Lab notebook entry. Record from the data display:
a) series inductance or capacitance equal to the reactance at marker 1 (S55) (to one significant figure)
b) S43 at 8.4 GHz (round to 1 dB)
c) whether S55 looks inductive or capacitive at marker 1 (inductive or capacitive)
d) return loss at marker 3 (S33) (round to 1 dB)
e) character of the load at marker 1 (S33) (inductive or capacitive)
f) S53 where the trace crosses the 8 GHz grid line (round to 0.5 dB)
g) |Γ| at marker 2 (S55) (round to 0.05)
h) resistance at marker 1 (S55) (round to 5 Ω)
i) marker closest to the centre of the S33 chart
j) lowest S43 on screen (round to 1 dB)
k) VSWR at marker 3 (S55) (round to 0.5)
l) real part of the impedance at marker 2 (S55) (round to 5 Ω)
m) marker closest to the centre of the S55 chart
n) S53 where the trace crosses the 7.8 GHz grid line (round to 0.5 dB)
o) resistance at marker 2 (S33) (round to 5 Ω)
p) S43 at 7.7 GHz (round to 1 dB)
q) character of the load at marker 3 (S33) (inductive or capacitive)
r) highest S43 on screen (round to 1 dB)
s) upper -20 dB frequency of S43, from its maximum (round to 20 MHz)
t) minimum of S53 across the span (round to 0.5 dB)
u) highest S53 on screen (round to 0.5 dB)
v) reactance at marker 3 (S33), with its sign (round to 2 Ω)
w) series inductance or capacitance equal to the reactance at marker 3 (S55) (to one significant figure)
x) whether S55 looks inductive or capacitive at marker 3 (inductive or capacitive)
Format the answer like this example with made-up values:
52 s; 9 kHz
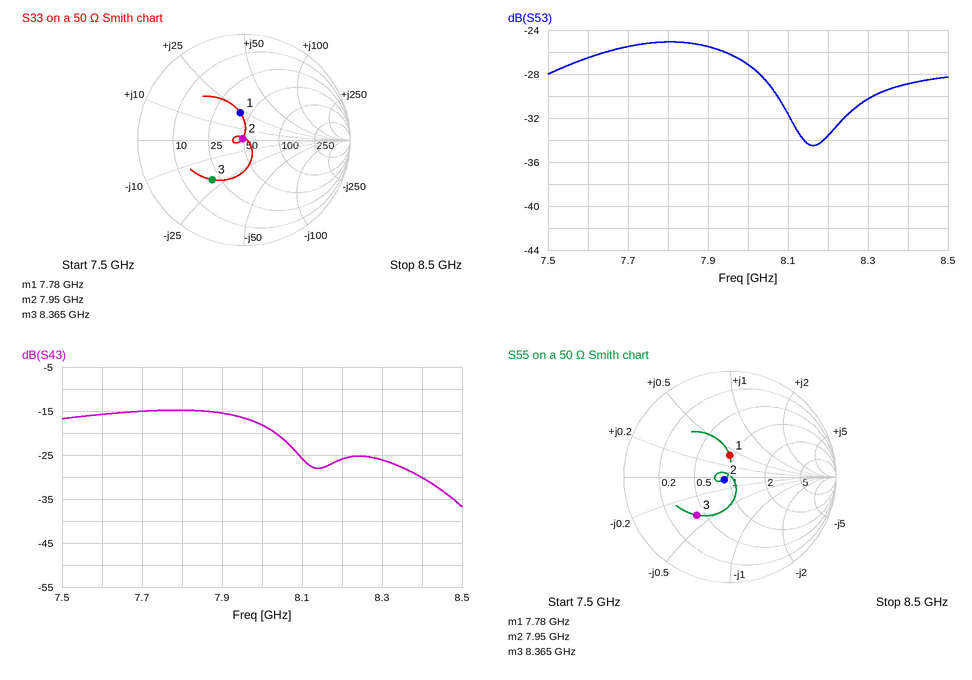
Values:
400 pH; -30 dB; inductive; 6 dB; inductive; -27.0 dB; 0.05; 45 Ω; marker 2; -37 dB; 3.0; 45 Ω; marker 2; -25.0 dB; 50 Ω; -15 dB; capacitive; -15 dB; 8.48 GHz; -34.5 dB; -25.0 dB; -20 Ω; 1.0 pF; capacitive
